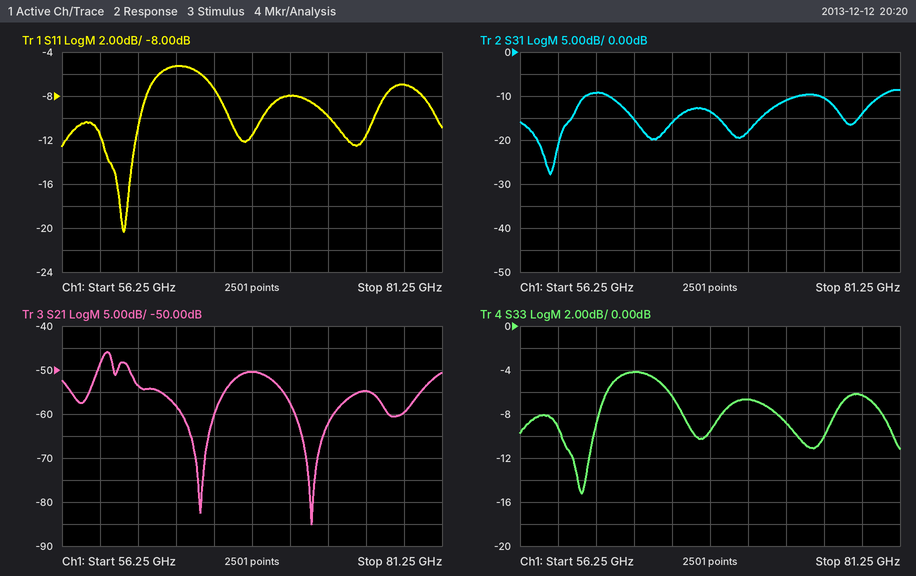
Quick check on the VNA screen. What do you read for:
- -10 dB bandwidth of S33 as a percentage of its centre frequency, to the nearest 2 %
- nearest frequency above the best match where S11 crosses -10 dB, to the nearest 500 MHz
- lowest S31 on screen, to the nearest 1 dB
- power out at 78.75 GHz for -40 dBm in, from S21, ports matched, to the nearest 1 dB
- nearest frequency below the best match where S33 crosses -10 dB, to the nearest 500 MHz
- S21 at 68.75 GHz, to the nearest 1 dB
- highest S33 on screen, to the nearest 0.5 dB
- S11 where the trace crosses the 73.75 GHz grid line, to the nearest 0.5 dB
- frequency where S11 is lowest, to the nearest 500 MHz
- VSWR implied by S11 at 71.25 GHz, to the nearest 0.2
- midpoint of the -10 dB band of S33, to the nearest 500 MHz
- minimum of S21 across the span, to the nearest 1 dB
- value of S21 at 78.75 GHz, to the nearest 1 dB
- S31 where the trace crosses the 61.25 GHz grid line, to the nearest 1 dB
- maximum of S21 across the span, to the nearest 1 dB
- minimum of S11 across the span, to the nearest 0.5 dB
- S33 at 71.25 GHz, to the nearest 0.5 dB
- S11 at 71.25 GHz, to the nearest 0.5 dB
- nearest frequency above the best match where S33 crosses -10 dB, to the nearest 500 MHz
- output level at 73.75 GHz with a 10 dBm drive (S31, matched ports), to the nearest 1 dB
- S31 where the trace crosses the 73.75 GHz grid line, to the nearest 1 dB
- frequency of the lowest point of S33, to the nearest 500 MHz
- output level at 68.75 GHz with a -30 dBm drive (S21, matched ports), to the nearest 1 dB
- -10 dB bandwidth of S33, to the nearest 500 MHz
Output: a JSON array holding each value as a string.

["4 %", "61.5 GHz", "-28 dB", "-100 dBm", "59.0 GHz", "-50 dB", "-4.0 dB", "-10.0 dB", "60.5 GHz", "2.4", "60.0 GHz", "-85 dB", "-60 dB", "-9 dB", "-46 dB", "-20.5 dB", "-6.5 dB", "-8.0 dB", "61.0 GHz", "-1 dBm", "-11 dB", "60.5 GHz", "-80 dBm", "2.0 GHz"]
